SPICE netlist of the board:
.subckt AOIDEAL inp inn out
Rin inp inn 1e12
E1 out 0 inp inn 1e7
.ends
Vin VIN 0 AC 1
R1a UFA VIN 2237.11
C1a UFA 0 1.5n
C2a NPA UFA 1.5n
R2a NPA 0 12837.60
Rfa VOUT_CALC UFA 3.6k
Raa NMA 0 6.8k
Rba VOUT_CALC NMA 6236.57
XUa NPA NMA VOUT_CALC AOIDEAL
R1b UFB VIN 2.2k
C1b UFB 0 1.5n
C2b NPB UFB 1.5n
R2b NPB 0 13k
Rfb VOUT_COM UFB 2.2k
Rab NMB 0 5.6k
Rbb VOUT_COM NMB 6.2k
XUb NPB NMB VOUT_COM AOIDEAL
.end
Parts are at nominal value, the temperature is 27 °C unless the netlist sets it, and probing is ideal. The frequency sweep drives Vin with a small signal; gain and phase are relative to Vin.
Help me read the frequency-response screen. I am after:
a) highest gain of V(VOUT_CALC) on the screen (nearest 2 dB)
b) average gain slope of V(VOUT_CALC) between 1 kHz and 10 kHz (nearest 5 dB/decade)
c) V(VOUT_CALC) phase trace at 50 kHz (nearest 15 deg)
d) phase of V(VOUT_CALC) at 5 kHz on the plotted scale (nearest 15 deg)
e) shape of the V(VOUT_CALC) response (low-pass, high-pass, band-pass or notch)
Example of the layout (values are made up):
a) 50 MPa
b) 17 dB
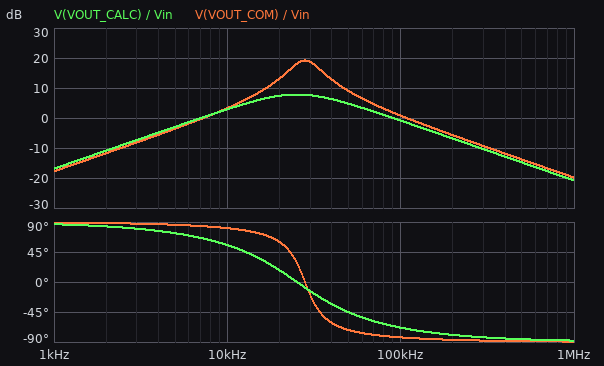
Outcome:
a) 8 dB
b) 20 dB/decade
c) -45 deg
d) 75 deg
e) band-pass
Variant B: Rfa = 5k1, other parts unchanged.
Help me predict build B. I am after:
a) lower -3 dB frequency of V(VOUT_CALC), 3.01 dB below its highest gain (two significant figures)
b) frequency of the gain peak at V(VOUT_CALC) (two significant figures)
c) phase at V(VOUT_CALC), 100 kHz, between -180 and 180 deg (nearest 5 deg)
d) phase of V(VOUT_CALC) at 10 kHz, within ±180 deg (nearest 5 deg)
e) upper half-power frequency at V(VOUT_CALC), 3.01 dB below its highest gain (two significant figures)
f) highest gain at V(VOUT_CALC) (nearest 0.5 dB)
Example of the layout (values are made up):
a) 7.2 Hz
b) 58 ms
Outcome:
a) 10 kHz
b) 24 kHz
c) -65 deg
d) 45 deg
e) 55 kHz
f) 6.0 dB
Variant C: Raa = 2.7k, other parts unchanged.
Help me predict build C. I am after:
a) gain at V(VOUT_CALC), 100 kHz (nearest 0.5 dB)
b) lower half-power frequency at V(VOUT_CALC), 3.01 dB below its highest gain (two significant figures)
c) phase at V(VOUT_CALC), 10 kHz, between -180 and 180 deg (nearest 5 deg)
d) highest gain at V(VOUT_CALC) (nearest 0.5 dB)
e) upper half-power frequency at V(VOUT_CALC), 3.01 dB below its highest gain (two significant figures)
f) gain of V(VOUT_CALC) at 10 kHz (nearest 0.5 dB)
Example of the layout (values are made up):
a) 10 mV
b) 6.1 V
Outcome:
a) 4.5 dB
b) 23 kHz
c) 95 deg
d) 31.5 dB
e) 27 kHz
f) 9.5 dB
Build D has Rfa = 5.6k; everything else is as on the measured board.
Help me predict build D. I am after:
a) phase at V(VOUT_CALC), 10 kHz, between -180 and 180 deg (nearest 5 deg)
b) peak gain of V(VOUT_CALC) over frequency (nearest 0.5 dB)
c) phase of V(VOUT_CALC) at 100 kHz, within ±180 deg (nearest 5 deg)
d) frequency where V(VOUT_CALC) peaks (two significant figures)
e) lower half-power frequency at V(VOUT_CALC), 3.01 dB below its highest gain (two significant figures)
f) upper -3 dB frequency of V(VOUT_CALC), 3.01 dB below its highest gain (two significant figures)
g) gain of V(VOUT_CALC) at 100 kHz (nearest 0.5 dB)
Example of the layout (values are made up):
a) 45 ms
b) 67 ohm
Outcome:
a) 45 deg
b) 6.0 dB
c) -65 deg
d) 23 kHz
e) 9.7 kHz
f) 56 kHz
g) -1.5 dB
